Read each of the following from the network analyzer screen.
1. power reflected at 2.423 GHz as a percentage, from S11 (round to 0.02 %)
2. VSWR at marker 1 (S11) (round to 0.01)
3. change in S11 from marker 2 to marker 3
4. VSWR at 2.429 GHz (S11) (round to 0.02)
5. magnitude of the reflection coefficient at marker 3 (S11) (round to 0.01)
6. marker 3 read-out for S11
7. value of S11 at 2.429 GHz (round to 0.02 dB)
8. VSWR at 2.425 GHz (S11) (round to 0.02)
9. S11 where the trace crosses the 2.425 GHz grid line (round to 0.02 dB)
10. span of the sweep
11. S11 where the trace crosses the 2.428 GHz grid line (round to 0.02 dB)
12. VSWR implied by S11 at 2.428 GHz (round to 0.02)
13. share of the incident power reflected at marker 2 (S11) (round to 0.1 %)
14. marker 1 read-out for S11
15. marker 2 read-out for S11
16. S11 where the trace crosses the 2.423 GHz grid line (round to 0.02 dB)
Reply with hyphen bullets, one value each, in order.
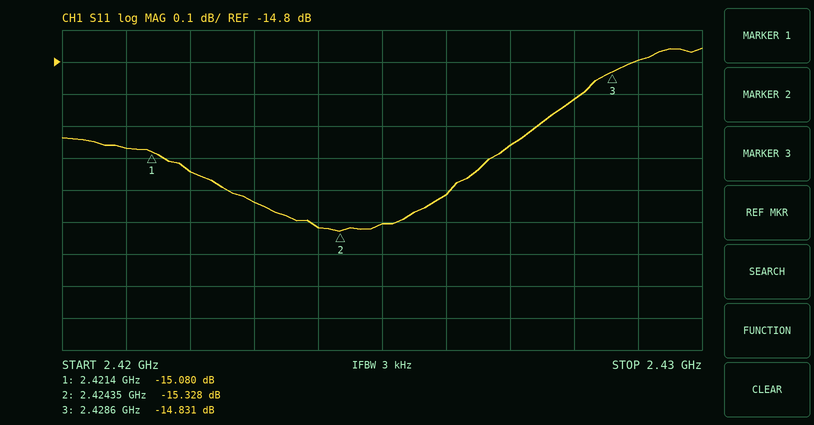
- 3.00 %
- 1.43
- 0.497 dB
- 1.44
- 0.18
- -14.831 dB
- -14.80 dB
- 1.42
- -15.30 dB
- 10 MHz
- -14.92 dB
- 1.44
- 2.9 %
- -15.080 dB
- -15.328 dB
- -15.24 dB
